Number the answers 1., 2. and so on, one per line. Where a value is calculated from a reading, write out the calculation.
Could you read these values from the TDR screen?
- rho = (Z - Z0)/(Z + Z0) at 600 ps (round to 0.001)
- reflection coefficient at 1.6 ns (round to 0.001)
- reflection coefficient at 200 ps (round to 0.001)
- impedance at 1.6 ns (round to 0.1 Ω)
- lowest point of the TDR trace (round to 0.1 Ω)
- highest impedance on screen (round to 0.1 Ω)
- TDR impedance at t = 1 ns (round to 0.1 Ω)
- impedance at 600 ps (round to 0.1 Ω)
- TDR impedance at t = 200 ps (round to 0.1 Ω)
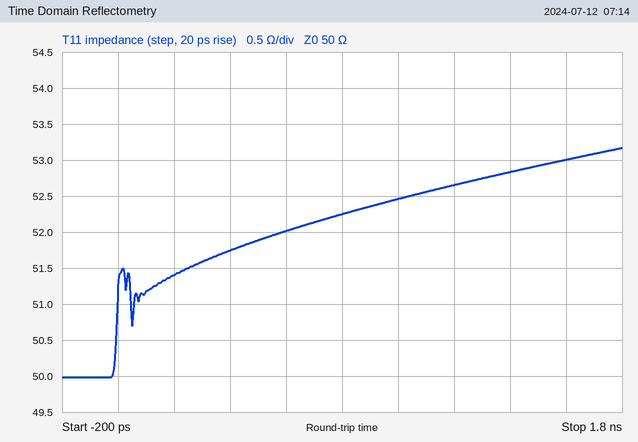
1. (52 − 50)/(52 + 50) ≈ +0.020
2. (53 − 50)/(53 + 50) ≈ +0.029
3. (51.4 − 50)/(51.4 + 50) ≈ +0.014
4. 53.0 Ω
5. 50.0 Ω
6. 53.2 Ω
7. 52.5 Ω
8. 52.0 Ω
9. 51.4 Ω
